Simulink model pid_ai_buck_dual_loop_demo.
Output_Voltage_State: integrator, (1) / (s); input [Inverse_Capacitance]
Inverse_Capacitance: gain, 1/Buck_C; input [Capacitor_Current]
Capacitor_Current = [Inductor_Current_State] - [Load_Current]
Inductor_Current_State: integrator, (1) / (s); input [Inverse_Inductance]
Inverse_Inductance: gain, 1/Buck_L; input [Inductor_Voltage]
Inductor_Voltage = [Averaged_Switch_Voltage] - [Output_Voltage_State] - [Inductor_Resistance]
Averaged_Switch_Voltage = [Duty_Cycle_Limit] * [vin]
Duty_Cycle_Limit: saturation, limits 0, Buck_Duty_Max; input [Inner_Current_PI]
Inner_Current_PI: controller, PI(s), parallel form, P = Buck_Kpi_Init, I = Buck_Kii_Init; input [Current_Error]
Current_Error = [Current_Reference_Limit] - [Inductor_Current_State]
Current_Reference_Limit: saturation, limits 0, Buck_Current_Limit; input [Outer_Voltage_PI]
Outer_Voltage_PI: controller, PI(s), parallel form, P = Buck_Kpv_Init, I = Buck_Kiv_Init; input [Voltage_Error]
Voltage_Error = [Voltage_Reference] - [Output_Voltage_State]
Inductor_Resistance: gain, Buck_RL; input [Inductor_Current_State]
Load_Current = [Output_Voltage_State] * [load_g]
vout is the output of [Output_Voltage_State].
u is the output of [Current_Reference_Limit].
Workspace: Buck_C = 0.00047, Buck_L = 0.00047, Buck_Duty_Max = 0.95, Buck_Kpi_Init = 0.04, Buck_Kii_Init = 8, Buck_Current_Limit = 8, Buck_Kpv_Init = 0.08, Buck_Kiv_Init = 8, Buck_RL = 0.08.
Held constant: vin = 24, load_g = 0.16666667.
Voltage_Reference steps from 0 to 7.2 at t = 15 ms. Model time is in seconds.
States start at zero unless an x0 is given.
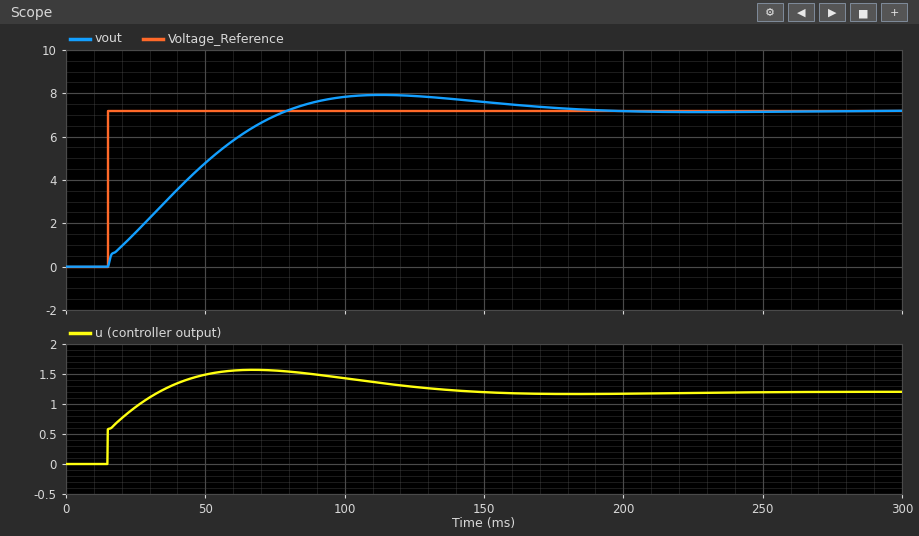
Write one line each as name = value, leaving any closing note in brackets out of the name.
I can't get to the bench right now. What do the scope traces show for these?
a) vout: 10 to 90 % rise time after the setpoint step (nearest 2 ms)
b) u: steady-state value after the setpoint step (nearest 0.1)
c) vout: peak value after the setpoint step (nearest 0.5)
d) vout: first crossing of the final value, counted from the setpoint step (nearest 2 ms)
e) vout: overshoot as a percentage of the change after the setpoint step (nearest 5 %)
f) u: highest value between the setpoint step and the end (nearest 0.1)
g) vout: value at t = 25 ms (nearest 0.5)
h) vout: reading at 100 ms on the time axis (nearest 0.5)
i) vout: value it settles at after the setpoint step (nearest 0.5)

vout: 10 to 90 % rise time after the setpoint step = 50 ms
u: steady-state value after the setpoint step = 1.2
vout: peak value after the setpoint step = 8.0
vout: first crossing of the final value, counted from the setpoint step = 64 ms
vout: overshoot as a percentage of the change after the setpoint step = 10 %
u: highest value between the setpoint step and the end = 1.6
vout: value at t = 25 ms = 1.5
vout: reading at 100 ms on the time axis = 8.0
vout: value it settles at after the setpoint step = 7.0
